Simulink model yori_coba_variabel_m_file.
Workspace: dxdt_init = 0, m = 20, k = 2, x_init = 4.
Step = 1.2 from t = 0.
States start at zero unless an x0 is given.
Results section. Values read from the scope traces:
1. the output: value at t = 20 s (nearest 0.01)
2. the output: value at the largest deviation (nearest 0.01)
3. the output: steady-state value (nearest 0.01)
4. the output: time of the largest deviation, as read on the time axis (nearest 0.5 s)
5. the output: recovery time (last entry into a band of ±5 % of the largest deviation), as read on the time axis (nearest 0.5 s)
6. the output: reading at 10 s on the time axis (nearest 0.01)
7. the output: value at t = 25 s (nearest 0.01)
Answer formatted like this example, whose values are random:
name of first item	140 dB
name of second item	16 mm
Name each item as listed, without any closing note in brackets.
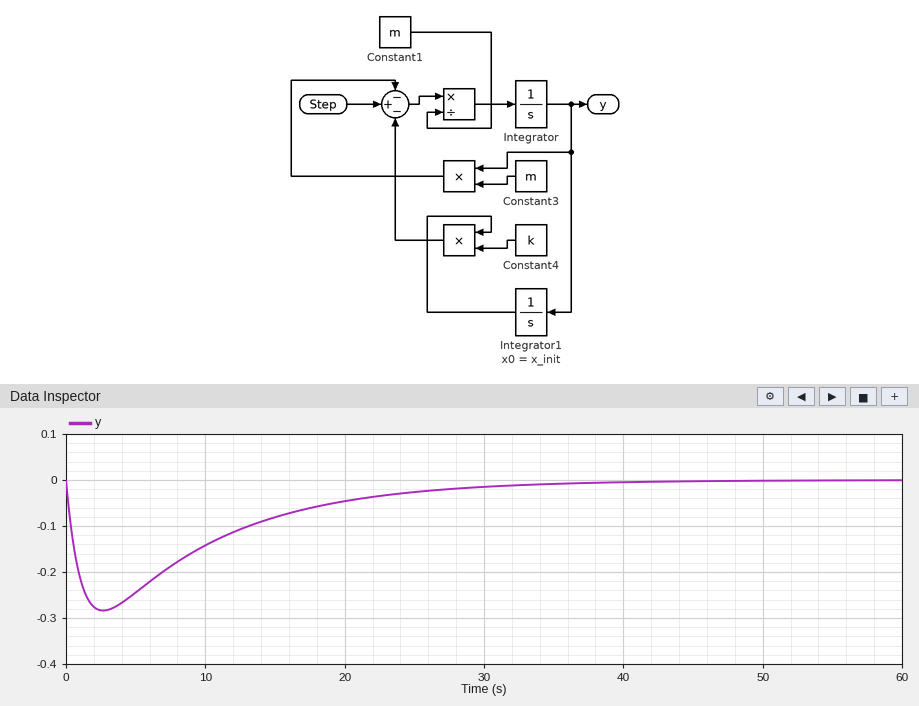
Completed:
the output: value at t = 20 s	-0.05
the output: value at the largest deviation	-0.28
the output: steady-state value	0.00
the output: time of the largest deviation, as read on the time axis	2.5 s
the output: recovery time (last entry into a band of ±5 % of the largest deviation), as read on the time axis	30.5 s
the output: reading at 10 s on the time axis	-0.14
the output: value at t = 25 s	-0.03
